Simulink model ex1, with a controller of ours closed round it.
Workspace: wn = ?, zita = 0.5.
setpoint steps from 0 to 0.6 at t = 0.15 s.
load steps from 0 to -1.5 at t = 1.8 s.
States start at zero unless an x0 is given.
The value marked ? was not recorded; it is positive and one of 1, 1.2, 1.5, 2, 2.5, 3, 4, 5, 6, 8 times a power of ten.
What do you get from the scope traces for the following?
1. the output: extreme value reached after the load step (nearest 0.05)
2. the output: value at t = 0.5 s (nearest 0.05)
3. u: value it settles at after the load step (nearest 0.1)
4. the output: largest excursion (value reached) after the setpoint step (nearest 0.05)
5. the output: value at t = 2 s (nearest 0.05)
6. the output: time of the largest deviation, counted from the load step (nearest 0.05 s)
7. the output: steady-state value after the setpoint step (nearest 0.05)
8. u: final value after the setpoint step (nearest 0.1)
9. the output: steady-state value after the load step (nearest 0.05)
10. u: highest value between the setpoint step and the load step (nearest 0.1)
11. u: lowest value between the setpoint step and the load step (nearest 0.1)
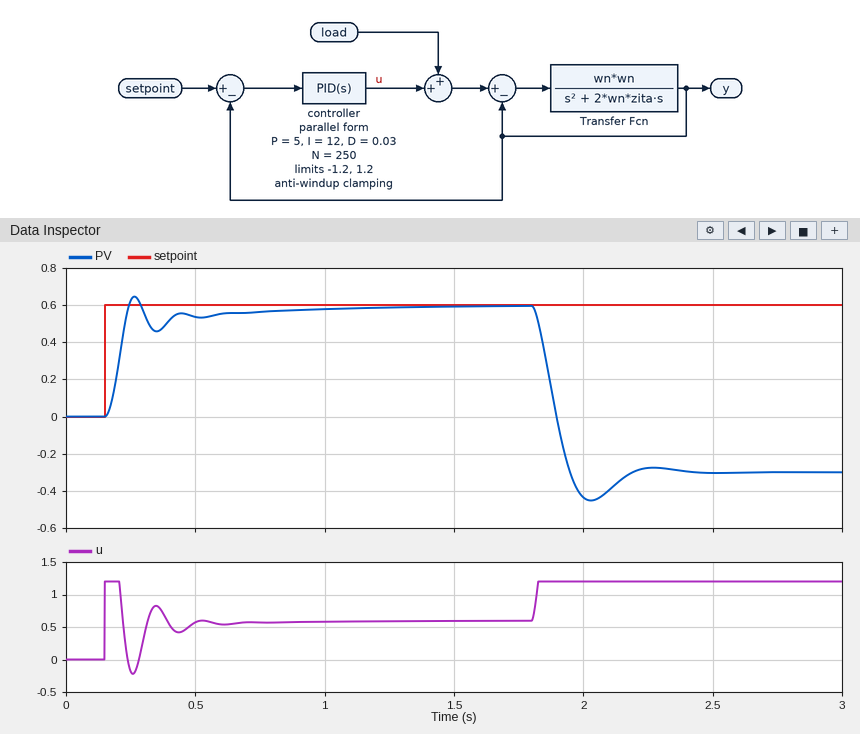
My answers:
-0.45
0.55
1.2
0.65
-0.45
0.25 s
0.60
0.6
-0.30
1.2
-0.2
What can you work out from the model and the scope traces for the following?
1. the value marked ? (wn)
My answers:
15
